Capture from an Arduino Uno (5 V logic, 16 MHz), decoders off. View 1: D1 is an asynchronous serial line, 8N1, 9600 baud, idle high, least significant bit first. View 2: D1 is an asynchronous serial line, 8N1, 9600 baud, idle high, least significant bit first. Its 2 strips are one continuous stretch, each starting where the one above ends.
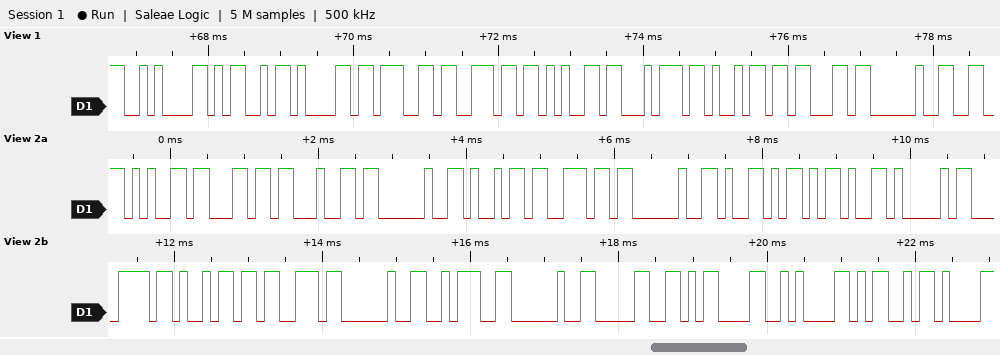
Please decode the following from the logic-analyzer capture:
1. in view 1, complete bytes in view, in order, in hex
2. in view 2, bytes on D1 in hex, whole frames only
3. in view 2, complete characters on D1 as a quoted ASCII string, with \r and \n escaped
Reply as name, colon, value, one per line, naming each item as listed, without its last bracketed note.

in view 1, complete bytes in view, in order, in hex: 0x0A 0x4D 0x61 0x67 0x6E 0x65 0x74 0x69 0x63 0x20
in view 2, bytes on D1 in hex, whole frames only: 65 6C 64 20 69 6E 20 59 2D 41 78 69 73 20 3A 20 30 0D 0A 4D
in view 2, complete characters on D1 as a quoted ASCII string, with \r and \n escaped: "eld in Y-Axis : 0\r\nM"
